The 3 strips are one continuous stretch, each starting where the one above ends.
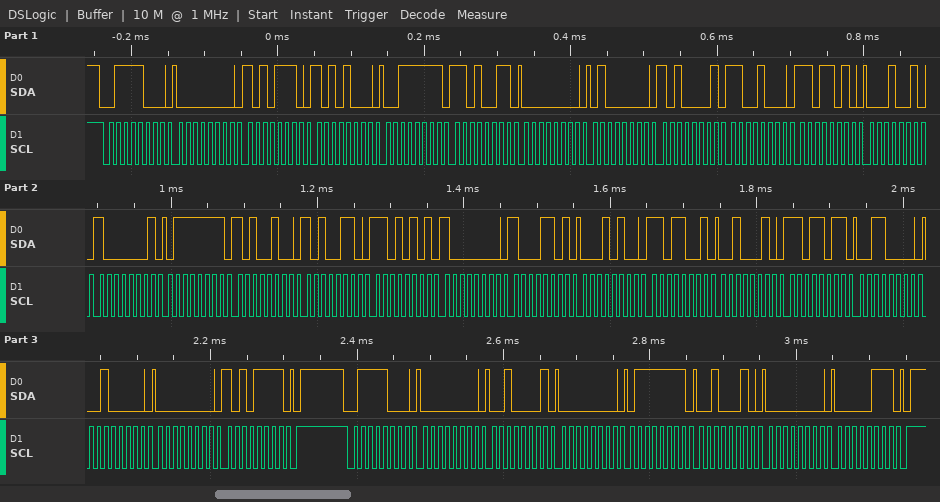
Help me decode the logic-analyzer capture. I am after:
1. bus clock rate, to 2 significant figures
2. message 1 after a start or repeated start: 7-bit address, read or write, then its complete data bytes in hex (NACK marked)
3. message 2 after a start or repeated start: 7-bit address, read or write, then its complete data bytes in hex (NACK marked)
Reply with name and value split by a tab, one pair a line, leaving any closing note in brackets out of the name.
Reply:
bus clock rate, to 2 significant figures	100 kHz
message 1 after a start or repeated start: 7-bit address, read or write, then its complete data bytes in hex	0x3C write: 00 AE A8 3F D3 00 40 A1 C8 DA 12 81 7F A4 A6 D5 80 8D 14 D9 22 DB 30 20 00 AF
message 2 after a start or repeated start: 7-bit address, read or write, then its complete data bytes in hex	0x3C write: 00 21 00 7F 22 00 07
